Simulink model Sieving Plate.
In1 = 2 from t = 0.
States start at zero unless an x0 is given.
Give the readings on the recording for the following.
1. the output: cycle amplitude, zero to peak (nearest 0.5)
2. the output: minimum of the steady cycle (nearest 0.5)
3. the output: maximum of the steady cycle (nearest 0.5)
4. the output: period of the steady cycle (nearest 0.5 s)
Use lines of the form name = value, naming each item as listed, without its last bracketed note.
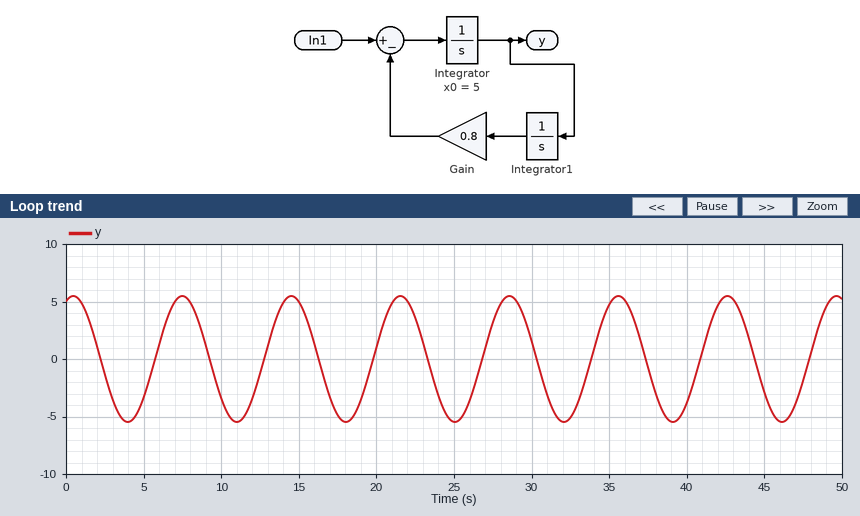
the output: cycle amplitude, zero to peak = 5.5
the output: minimum of the steady cycle = -5.5
the output: maximum of the steady cycle = 5.5
the output: period of the steady cycle = 7.0 s
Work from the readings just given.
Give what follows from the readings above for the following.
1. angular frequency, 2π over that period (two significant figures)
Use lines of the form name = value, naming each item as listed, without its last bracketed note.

angular frequency, 2π over that period = 0.90 rad/s
